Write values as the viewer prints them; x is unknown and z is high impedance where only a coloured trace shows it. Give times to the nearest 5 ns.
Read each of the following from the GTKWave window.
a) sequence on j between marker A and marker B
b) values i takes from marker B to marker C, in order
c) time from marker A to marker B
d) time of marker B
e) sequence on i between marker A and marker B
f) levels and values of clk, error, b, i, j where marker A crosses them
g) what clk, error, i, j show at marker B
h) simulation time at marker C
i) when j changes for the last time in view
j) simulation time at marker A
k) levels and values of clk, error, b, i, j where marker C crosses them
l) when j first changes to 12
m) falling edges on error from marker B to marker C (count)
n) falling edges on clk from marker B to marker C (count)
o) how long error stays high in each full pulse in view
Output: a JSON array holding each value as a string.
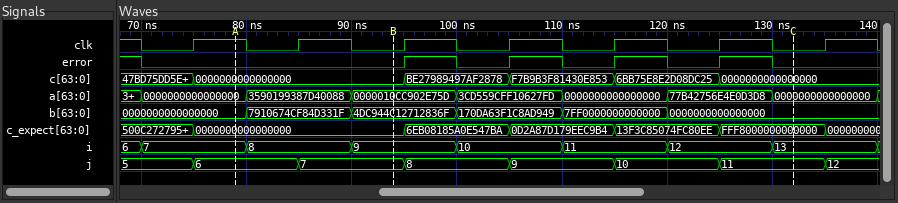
["6, 7", "9, 10, 11, 12, 13", "15 ns", "95 ns", "7, 8, 9", "clk=1, error=0, b=0000000000000000, i=7, j=6", "clk=0, error=0, i=9, j=7", "130 ns", "135 ns", "80 ns", "clk=0, error=0, b=0000000000000000, i=13, j=11", "135 ns", "4", "4", "5 ns, 5 ns, 5 ns, 5 ns"]
